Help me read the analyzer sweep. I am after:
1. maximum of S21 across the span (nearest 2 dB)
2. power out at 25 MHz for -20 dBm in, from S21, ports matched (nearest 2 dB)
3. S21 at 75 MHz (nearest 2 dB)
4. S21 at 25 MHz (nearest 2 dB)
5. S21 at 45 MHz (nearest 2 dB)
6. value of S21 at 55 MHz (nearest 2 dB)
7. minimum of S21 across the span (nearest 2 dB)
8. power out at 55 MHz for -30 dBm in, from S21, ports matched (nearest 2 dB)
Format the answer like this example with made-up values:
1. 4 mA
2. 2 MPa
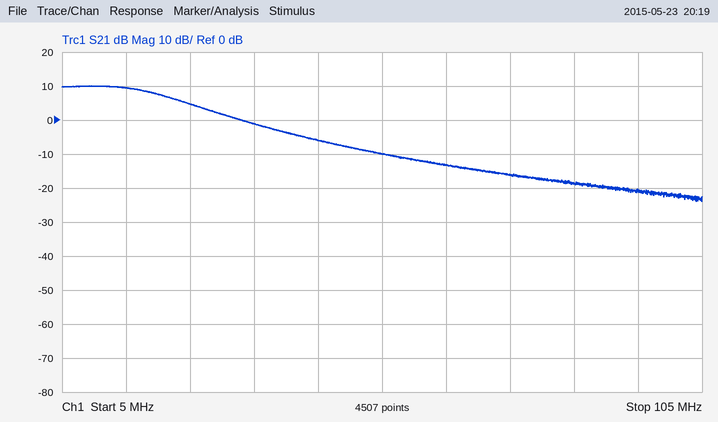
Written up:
1. 10 dB
2. -16 dBm
3. -16 dB
4. 4 dB
5. -6 dB
6. -10 dB
7. -24 dB
8. -40 dBm
